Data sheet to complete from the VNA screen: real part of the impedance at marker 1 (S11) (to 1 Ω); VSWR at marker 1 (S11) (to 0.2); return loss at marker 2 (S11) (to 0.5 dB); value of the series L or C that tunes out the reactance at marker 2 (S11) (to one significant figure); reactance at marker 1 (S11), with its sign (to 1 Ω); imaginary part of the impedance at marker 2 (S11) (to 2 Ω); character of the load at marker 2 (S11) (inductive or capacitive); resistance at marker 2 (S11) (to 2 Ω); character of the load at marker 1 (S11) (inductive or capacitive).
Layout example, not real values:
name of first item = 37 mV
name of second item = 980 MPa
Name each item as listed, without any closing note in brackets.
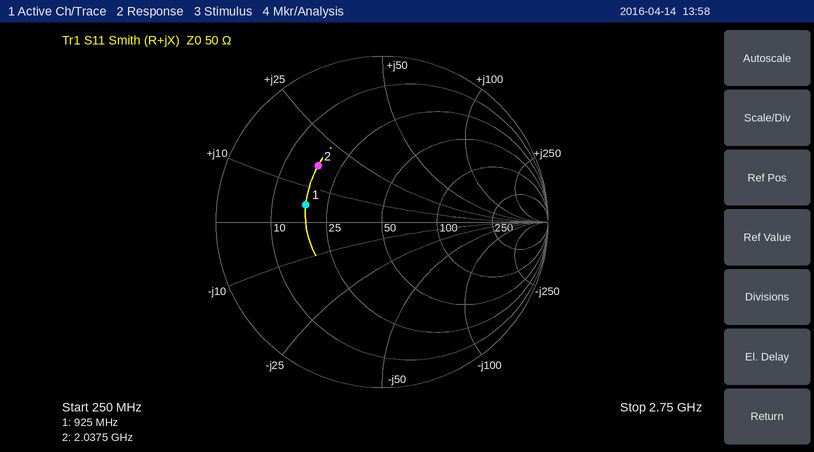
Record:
real part of the impedance at marker 1 (S11) = 18 Ω
VSWR at marker 1 (S11) = 2.8
return loss at marker 2 (S11) = 6.0 dB
value of the series L or C that tunes out the reactance at marker 2 (S11) = 5 pF
reactance at marker 1 (S11), with its sign = +5 Ω
imaginary part of the impedance at marker 2 (S11) = +16 Ω
character of the load at marker 2 (S11) = inductive
resistance at marker 2 (S11) = 18 Ω
character of the load at marker 1 (S11) = inductive
